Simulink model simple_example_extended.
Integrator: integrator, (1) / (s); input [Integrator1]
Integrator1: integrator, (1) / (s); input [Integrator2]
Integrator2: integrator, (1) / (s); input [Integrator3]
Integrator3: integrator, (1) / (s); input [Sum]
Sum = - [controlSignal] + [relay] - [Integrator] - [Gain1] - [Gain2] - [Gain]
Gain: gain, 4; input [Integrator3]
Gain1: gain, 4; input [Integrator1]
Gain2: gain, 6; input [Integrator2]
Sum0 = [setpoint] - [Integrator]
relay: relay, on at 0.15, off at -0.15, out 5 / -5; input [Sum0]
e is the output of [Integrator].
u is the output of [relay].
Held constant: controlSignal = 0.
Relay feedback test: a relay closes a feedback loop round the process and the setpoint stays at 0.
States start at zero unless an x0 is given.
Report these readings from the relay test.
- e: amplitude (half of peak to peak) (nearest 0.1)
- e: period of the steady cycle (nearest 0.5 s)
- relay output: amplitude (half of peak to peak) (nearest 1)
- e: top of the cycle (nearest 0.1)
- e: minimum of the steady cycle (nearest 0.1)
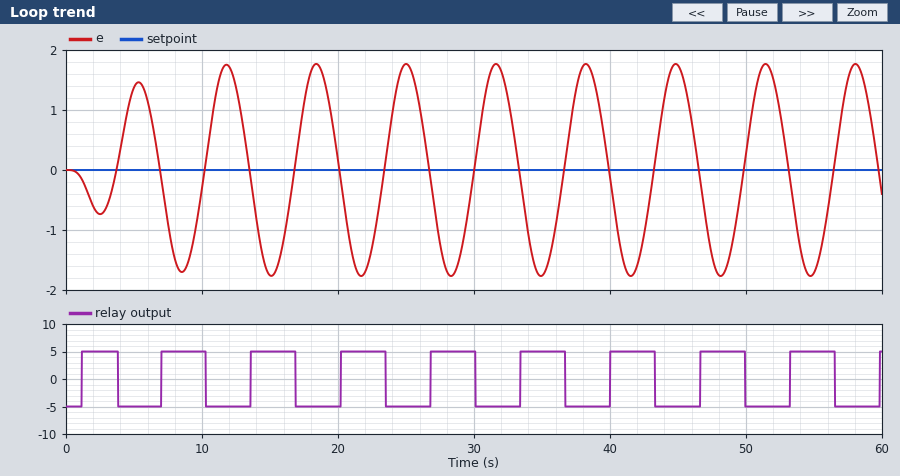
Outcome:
1.8
6.5 s
5
1.8
-1.8
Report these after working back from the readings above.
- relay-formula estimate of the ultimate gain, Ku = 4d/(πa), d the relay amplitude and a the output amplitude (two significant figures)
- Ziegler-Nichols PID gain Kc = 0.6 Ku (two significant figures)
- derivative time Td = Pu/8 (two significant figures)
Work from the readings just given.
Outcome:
3.5
2.1
0.81 s
